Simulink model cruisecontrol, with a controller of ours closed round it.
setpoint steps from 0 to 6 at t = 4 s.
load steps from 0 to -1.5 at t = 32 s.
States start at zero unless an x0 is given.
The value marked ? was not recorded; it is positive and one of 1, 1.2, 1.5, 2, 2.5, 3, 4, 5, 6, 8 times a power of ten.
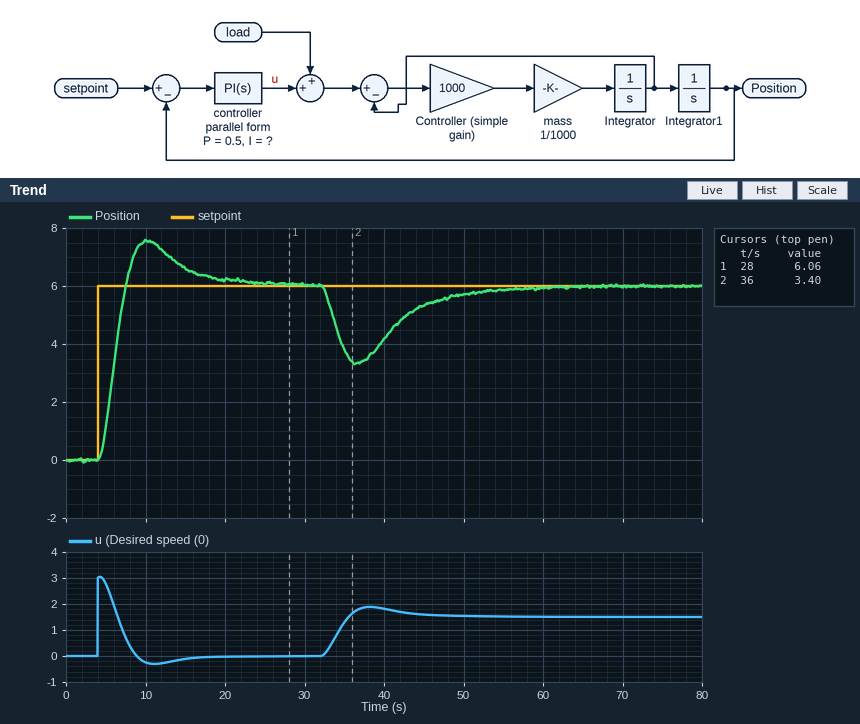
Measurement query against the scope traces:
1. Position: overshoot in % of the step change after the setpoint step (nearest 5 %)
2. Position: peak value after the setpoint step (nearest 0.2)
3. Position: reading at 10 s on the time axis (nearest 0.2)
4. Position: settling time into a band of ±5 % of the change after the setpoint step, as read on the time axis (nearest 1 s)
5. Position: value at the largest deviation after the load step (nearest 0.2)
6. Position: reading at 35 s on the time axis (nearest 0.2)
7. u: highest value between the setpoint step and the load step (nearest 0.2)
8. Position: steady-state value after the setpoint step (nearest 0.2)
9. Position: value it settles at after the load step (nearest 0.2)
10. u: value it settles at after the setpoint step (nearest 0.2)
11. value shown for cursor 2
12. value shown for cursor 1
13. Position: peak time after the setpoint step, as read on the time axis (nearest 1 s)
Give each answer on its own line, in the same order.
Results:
25 %
7.6
7.6
18 s
3.4
3.8
3.0
6.0
6.0
0.0
3.40
6.06
10 s
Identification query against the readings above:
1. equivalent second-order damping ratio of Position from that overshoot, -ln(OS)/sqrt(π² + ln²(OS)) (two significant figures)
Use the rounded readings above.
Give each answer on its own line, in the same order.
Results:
0.40
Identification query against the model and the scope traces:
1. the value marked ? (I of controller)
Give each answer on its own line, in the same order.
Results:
0.06
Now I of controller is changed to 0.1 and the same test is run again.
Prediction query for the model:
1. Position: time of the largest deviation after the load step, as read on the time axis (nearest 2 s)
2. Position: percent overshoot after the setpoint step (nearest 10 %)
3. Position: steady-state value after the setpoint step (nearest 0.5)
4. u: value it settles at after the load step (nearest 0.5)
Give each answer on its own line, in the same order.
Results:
36 s
40 %
6.0
1.5
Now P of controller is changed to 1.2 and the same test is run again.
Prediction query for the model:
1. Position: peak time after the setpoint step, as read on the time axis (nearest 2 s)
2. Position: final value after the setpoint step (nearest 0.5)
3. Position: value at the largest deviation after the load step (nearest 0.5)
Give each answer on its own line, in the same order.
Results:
8 s
6.0
4.5
